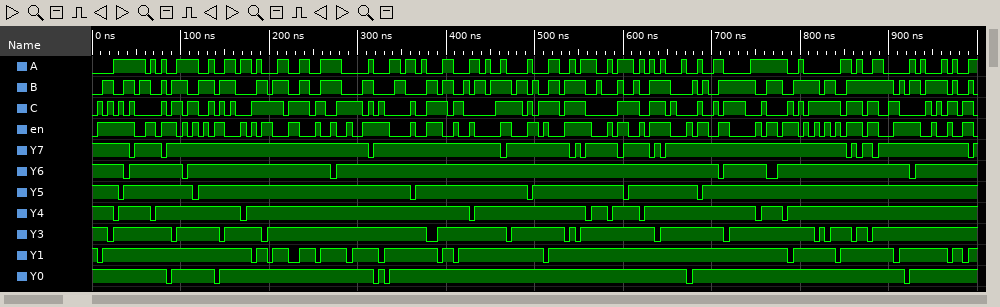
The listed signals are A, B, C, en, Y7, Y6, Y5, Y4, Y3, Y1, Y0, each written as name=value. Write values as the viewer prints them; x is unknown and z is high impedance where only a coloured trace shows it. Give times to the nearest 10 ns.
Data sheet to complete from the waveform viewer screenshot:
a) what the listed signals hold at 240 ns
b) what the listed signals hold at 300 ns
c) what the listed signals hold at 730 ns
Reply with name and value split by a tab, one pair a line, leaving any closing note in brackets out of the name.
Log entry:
what the listed signals hold at 240 ns	A=1, B=1, C=1, en=0, Y7=1, Y6=1, Y5=1, Y4=1, Y3=1, Y1=1, Y0=1
what the listed signals hold at 300 ns	A=0, B=0, C=1, en=0, Y7=1, Y6=1, Y5=1, Y4=1, Y3=1, Y1=1, Y0=1
what the listed signals hold at 730 ns	A=0, B=1, C=1, en=0, Y7=1, Y6=1, Y5=1, Y4=1, Y3=1, Y1=1, Y0=1
